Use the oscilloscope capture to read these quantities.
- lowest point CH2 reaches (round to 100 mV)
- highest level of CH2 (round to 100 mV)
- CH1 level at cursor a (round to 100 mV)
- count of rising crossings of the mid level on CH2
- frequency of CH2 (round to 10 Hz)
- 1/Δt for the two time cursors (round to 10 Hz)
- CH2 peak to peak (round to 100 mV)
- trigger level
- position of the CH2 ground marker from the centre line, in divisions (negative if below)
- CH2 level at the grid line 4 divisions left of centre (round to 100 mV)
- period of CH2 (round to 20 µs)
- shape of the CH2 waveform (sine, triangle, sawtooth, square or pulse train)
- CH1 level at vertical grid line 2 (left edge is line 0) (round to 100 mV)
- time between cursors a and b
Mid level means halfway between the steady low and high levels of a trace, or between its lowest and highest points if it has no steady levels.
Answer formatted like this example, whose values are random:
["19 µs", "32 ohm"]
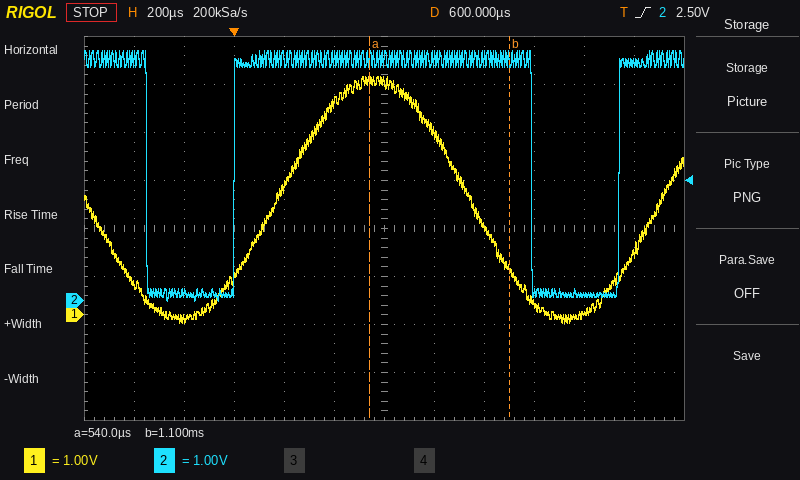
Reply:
["0.0 V", "5.2 V", "4.9 V", "2", "650 Hz", "1.79 kHz", "5.2 V", "2.50 V", "-1.5 div", "200 mV", "1.54 ms", "pulse train", "-100 mV", "560 µs"]
